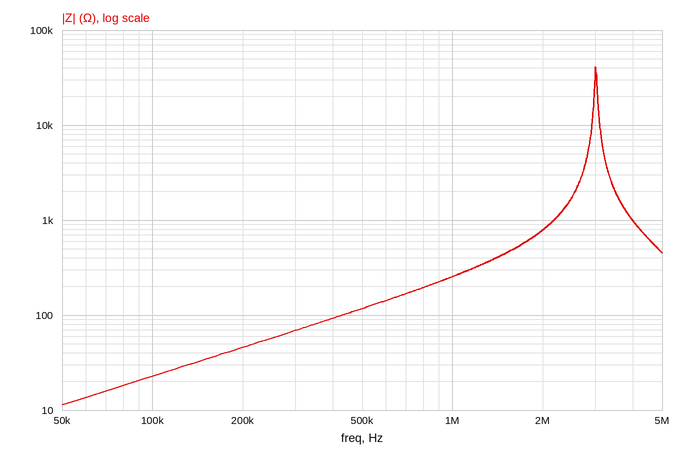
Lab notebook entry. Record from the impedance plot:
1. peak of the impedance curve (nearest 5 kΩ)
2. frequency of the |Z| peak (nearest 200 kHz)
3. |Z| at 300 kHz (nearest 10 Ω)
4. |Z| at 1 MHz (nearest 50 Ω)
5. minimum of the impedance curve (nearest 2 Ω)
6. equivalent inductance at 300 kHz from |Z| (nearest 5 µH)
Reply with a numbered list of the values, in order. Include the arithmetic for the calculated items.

1. 40 kΩ
2. 3.0 MHz
3. 70 Ω
4. 250 Ω
5. 12 Ω
6. L = 70 Ω/(2π × 300 kHz) ≈ 37.1 µH, so 35 µH to the nearest 5 µH
